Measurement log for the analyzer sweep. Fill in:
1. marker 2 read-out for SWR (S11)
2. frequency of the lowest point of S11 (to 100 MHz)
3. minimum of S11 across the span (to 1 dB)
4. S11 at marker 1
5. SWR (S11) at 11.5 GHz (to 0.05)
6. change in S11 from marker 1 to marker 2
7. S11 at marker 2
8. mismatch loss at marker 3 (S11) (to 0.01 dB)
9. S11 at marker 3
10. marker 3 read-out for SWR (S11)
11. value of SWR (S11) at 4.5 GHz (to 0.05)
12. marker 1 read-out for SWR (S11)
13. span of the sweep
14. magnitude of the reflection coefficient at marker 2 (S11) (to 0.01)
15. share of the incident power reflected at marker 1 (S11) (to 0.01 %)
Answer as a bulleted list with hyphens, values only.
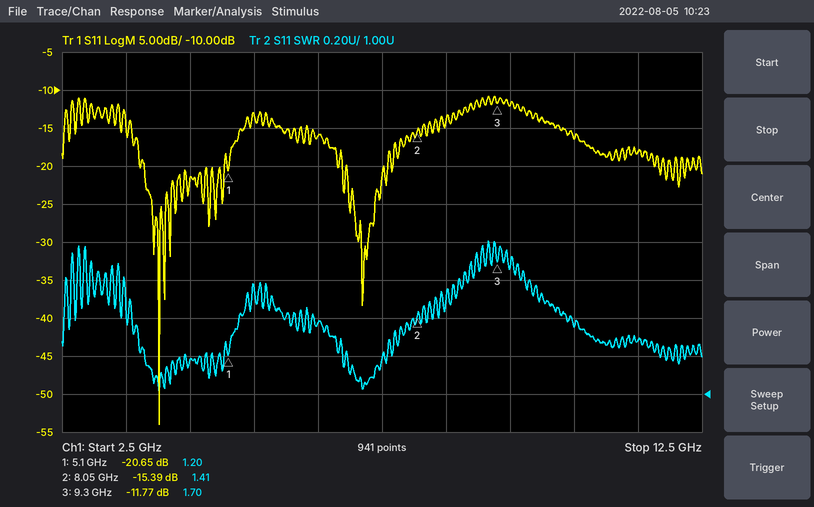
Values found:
- 1.41
- 4.0 GHz
- -54 dB
- -20.65 dB
- 1.30
- 5.26 dB
- -15.39 dB
- 0.30 dB
- -11.77 dB
- 1.70
- 1.20
- 1.20
- 10 GHz
- 0.17
- 0.86 %
